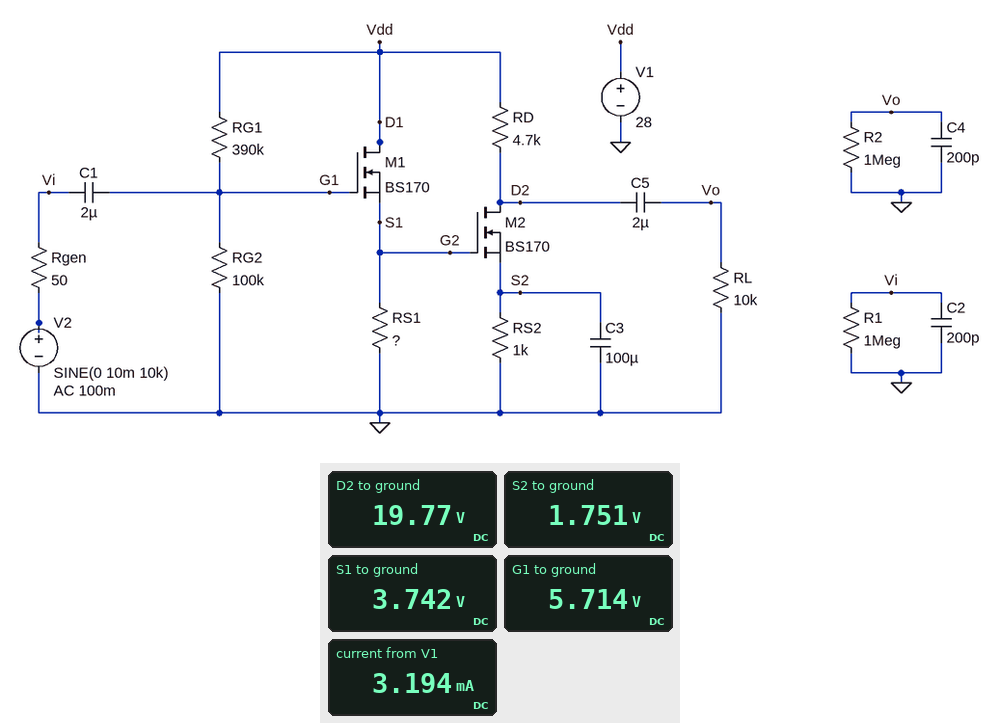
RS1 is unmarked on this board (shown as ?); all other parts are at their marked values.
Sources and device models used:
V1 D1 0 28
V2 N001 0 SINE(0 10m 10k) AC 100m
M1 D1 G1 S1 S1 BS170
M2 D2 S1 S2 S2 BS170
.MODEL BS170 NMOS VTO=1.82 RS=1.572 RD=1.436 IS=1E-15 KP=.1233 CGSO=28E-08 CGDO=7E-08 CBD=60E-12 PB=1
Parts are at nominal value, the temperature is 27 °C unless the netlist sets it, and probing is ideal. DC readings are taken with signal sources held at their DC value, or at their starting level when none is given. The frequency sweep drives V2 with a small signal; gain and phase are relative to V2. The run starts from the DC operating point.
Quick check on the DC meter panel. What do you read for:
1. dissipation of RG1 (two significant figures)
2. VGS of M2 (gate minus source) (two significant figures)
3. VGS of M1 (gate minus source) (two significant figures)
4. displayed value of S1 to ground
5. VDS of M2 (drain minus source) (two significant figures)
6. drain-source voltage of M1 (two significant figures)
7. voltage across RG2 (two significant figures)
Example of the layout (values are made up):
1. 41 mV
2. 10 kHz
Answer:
1. 1.3 mW
2. 2.0 V
3. 2.0 V
4. 3.742 V
5. 18 V
6. 24 V
7. 5.7 V
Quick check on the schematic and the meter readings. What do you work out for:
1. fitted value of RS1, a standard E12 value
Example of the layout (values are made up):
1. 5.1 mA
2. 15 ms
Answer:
1. 2.7 kΩ
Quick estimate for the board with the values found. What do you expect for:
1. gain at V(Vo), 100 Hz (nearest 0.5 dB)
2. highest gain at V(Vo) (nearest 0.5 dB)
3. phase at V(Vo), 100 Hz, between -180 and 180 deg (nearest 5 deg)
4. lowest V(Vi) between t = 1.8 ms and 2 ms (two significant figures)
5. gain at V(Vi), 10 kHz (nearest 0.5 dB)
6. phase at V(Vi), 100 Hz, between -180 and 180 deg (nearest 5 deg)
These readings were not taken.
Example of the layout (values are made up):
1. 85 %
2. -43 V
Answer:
1. 35.5 dB
2. 36.0 dB
3. -160 deg
4. -10 mV
5. 0 dB
6. 0 deg
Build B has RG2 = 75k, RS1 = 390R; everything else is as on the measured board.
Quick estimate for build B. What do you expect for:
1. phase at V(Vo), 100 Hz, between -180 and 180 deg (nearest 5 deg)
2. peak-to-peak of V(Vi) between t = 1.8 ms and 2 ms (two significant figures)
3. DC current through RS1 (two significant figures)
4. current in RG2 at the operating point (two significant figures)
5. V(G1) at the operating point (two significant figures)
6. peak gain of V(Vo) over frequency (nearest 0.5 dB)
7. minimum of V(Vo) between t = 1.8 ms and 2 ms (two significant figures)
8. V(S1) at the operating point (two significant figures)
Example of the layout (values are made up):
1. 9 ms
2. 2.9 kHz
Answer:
1. -165 deg
2. 20 mV
3. 6.1 mA
4. 60 µA
5. 4.5 V
6. 30.0 dB
7. -330 mV
8. 2.4 V
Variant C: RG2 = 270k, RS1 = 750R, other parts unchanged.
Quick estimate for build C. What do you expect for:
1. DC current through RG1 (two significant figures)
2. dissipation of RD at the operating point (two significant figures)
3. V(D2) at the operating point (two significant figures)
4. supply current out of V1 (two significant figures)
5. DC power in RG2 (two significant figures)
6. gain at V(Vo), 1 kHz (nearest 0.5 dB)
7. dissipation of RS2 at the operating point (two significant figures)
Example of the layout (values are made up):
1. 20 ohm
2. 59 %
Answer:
1. 42 µA
2. 110 mW
3. 4.9 V
4. 17 mA
5. 490 µW
6. -43.5 dB
7. 24 mW
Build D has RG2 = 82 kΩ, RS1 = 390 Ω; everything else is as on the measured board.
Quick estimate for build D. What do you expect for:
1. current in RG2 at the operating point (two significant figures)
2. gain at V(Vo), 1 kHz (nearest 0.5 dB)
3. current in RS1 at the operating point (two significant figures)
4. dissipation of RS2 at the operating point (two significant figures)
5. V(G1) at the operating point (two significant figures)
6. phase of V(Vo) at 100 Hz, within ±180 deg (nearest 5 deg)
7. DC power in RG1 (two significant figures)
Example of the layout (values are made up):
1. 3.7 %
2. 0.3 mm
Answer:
1. 59 µA
2. 32.0 dB
3. 6.9 mA
4. 590 µW
5. 4.9 V
6. -165 deg
7. 1.4 mW
